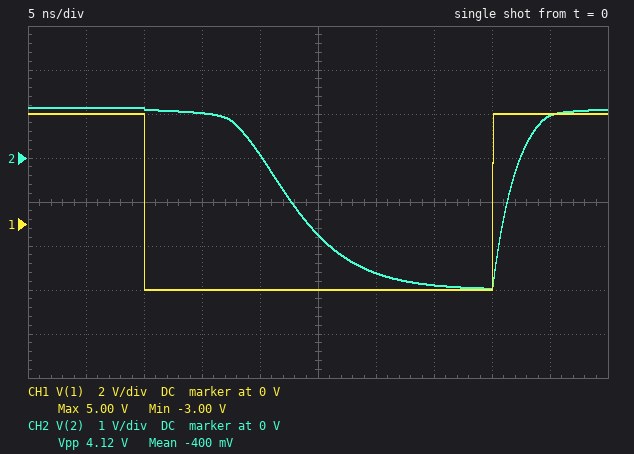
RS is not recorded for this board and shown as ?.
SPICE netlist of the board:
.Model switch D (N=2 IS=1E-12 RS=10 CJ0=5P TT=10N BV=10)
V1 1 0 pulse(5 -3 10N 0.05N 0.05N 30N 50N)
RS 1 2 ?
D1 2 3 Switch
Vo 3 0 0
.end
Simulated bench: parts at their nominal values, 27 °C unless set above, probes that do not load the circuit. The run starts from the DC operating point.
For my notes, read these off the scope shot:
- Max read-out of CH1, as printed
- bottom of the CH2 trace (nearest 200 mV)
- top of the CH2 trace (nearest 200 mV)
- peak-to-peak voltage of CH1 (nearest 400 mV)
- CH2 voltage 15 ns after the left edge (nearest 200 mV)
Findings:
5.00 V
-3.0 V
1.2 V
8.0 V
1.0 V
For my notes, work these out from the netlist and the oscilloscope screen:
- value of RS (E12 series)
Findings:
1.5 kΩ
